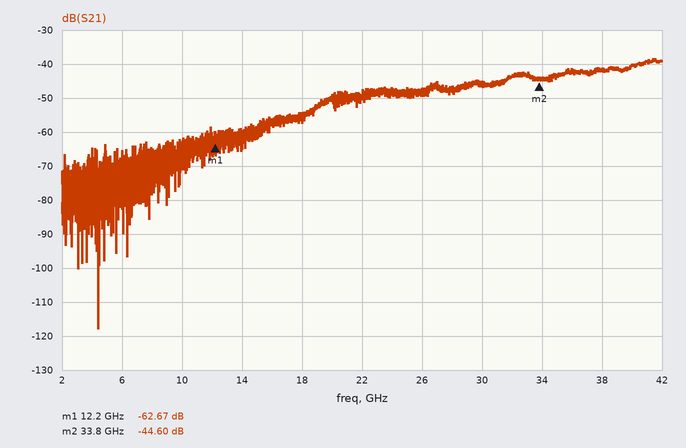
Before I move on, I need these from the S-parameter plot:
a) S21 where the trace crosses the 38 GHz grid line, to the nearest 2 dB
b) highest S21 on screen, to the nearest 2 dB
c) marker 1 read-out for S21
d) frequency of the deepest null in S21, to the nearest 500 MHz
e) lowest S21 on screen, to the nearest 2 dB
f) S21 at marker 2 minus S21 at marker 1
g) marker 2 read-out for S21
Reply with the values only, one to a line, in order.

-42 dB
-38 dB
-62.67 dB
4.5 GHz
-118 dB
18.07 dB
-44.60 dB
